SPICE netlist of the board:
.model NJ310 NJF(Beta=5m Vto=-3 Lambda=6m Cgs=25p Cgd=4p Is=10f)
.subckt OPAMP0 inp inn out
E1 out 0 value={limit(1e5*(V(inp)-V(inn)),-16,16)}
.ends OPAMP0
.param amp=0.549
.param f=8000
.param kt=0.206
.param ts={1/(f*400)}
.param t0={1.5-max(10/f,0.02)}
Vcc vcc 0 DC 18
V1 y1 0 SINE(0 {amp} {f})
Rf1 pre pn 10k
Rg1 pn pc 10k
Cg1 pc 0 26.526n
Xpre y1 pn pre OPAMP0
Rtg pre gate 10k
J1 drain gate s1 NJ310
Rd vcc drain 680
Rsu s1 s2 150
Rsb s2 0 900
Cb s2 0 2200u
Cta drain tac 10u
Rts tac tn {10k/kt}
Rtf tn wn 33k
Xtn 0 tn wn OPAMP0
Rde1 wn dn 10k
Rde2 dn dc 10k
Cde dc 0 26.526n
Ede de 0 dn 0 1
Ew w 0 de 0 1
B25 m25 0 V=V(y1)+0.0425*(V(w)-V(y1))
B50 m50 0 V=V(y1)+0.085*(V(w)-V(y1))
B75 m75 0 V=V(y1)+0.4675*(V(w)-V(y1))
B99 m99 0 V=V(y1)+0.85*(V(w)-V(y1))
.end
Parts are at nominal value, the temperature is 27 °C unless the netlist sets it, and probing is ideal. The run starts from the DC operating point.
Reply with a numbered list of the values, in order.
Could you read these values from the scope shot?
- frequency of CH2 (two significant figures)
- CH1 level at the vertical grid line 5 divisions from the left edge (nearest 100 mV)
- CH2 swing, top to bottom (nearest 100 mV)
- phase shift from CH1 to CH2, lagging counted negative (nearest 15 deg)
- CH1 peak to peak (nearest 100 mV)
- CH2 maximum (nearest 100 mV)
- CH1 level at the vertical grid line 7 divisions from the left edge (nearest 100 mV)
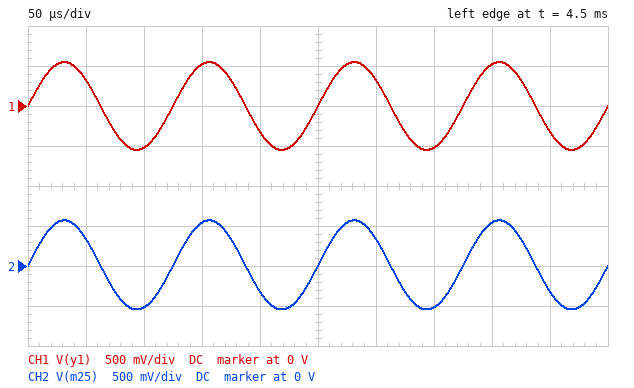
1. 8.0 kHz
2. 0 V
3. 1.1 V
4. 0 deg
5. 1.1 V
6. 600 mV
7. -500 mV
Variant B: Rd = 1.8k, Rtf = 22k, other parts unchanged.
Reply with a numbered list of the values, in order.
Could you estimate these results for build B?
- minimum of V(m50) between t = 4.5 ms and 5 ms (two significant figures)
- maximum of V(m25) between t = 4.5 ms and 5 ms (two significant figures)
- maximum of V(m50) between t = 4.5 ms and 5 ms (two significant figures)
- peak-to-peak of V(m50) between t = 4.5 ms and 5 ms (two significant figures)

1. -560 mV
2. 600 mV
3. 660 mV
4. 1.2 V
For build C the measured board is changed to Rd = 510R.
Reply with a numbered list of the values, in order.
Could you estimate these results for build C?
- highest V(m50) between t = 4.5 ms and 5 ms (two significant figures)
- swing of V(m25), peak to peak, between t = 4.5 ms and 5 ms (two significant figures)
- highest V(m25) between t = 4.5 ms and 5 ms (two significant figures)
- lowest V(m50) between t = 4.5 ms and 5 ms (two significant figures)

1. 570 mV
2. 1.1 V
3. 560 mV
4. -530 mV
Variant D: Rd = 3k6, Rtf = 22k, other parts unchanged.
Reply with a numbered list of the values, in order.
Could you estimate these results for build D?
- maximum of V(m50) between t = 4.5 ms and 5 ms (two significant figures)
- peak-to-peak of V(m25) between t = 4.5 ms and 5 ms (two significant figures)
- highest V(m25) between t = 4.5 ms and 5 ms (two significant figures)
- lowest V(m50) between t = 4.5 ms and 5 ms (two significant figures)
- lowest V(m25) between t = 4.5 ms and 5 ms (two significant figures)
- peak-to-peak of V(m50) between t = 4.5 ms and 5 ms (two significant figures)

1. 640 mV
2. 1.2 V
3. 590 mV
4. -650 mV
5. -600 mV
6. 1.3 V
